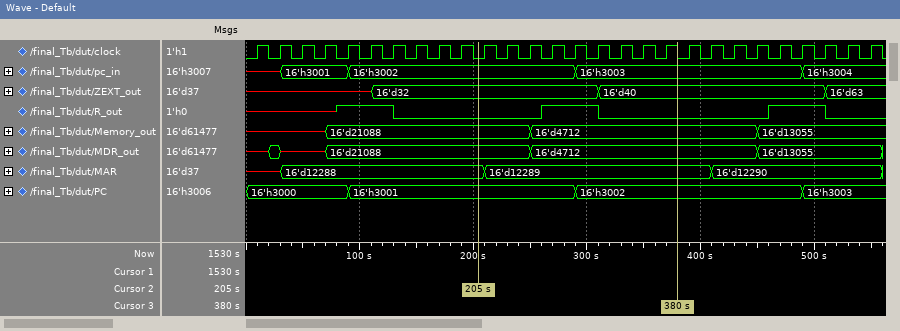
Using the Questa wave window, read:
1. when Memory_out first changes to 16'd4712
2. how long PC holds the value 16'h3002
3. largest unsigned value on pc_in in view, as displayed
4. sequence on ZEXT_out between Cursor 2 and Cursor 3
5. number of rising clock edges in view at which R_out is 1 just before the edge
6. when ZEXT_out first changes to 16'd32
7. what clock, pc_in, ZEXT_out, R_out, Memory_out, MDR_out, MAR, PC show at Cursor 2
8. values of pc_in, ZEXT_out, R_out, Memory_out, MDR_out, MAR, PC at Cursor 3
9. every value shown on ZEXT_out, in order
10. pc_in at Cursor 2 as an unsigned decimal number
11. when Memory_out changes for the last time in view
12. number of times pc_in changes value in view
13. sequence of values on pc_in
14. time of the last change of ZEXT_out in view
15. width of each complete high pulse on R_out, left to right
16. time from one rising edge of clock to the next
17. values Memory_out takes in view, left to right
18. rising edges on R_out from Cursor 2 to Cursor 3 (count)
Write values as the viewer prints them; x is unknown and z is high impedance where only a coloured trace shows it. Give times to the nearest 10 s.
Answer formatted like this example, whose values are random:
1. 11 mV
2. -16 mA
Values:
1. 250 s
2. 200 s
3. 16'h3004
4. 16'd32, 16'd40
5. 9
6. 110 s
7. clock=0, pc_in=16'h3002, ZEXT_out=16'd32, R_out=0, Memory_out=16'd21088, MDR_out=16'd21088, MAR=16'd12288, PC=16'h3001
8. pc_in=16'h3003, ZEXT_out=16'd40, R_out=0, Memory_out=16'd4712, MDR_out=16'd4712, MAR=16'd12289, PC=16'h3002
9. x, 16'd32, 16'd40, 16'd63
10. 12290
11. 450 s
12. 4
13. x, 16'h3001, 16'h3002, 16'h3003, 16'h3004
14. 510 s
15. 50 s, 50 s
16. 20 s
17. x, 16'd21088, 16'd4712, 16'd13055
18. 1
